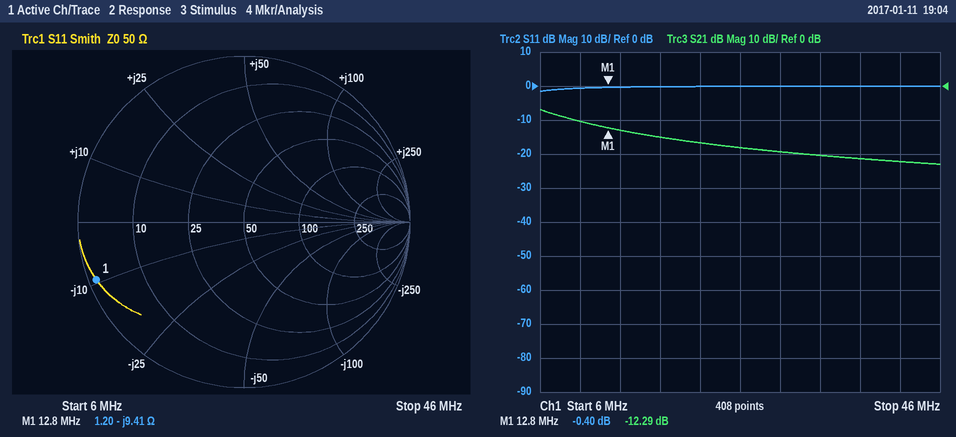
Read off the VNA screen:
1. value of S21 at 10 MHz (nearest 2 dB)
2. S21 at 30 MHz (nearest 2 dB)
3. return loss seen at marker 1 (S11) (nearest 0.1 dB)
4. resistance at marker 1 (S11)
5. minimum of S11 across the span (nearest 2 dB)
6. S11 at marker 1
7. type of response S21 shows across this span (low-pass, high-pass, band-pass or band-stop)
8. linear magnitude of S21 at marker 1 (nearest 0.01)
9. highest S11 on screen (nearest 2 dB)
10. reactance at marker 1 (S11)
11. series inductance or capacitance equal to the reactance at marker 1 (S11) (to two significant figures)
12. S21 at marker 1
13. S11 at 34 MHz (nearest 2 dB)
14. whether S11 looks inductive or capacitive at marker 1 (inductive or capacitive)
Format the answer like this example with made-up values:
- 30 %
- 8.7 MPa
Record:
- -10 dB
- -20 dB
- 0.4 dB
- 1.20 Ω
- -2 dB
- -0.40 dB
- low-pass
- 0.24
- 0 dB
- -9.41 Ω
- 1.3 nF
- -12.29 dB
- 0 dB
- capacitive
